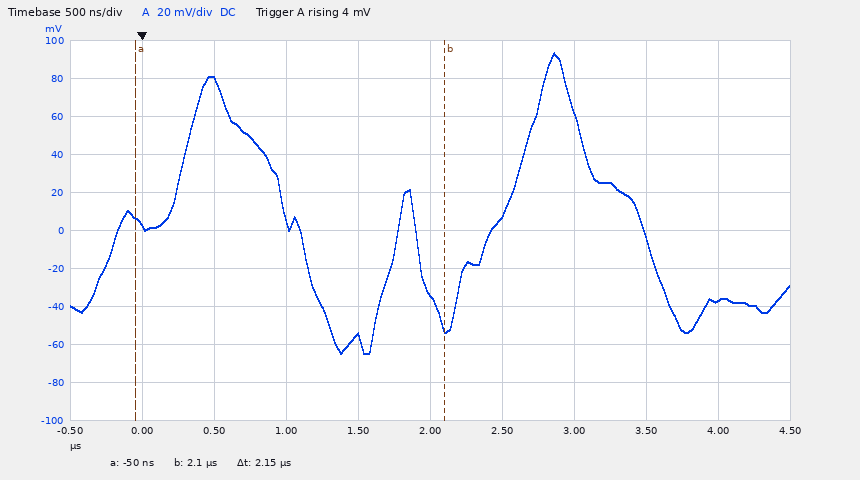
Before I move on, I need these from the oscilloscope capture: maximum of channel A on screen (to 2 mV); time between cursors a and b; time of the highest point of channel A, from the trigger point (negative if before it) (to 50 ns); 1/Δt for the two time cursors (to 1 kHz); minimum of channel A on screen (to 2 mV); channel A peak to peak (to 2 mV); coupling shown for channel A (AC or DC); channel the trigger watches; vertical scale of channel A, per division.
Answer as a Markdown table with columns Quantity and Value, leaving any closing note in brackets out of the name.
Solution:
| Quantity | Value |
|---|---|
| maximum of channel A on screen | 94 mV |
| time between cursors a and b | 2.15 µs |
| time of the highest point of channel A, from the trigger point (negative if before it) | +2.85 µs |
| 1/Δt for the two time cursors | 465 kHz |
| minimum of channel A on screen | -64 mV |
| channel A peak to peak | 158 mV |
| coupling shown for channel A | DC |
| channel the trigger watches | channel A |
| vertical scale of channel A, per division | 20 mV |
